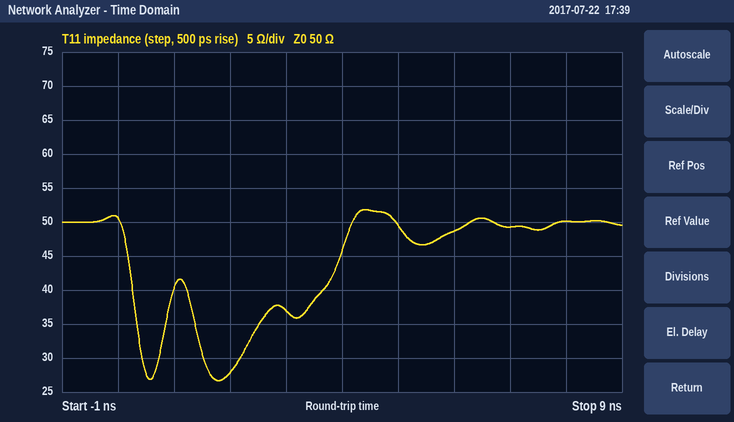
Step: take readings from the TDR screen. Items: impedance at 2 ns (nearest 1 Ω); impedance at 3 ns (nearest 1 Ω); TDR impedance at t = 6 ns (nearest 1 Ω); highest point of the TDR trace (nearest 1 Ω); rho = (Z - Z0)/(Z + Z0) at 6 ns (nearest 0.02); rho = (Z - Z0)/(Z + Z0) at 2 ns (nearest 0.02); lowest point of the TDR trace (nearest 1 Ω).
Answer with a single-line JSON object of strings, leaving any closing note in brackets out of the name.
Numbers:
{"impedance at 2 ns": "28 Ω", "impedance at 3 ns": "37 Ω", "TDR impedance at t = 6 ns": "49 Ω", "highest point of the TDR trace": "52 Ω", "rho = (Z - Z0)/(Z + Z0) at 6 ns": "-0.02", "rho = (Z - Z0)/(Z + Z0) at 2 ns": "-0.28", "lowest point of the TDR trace": "27 Ω"}
